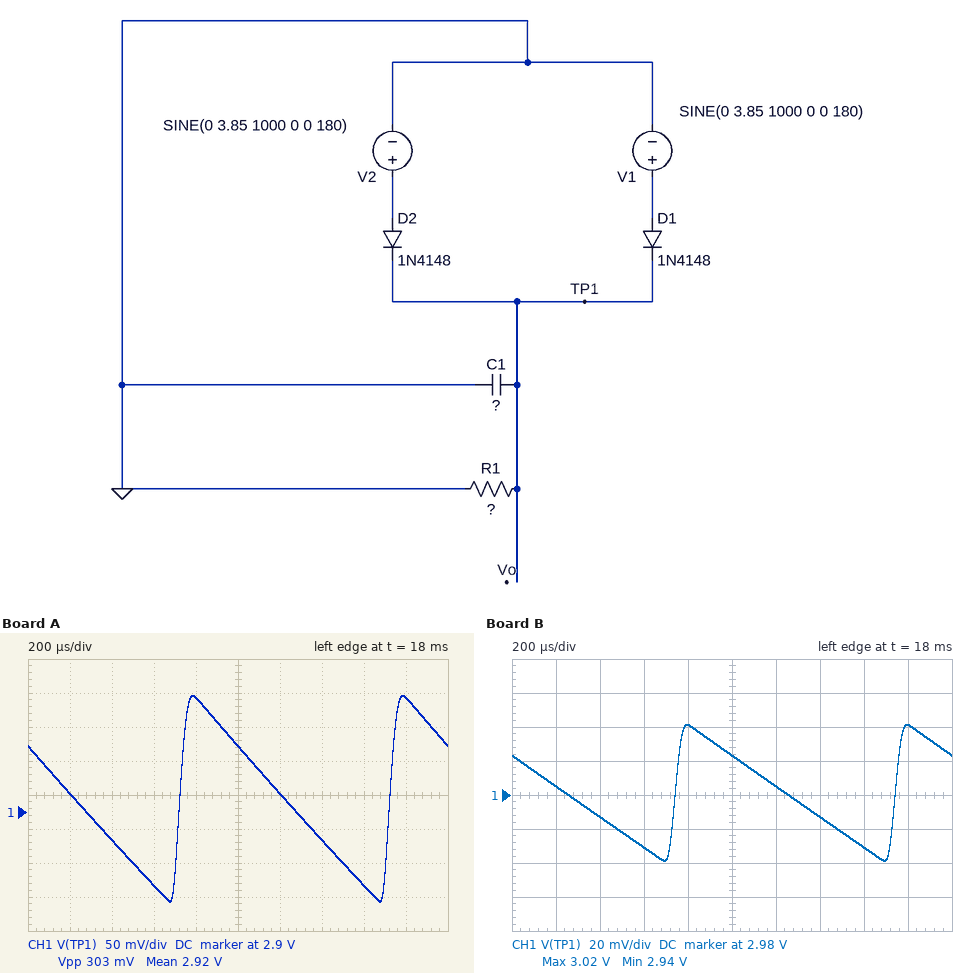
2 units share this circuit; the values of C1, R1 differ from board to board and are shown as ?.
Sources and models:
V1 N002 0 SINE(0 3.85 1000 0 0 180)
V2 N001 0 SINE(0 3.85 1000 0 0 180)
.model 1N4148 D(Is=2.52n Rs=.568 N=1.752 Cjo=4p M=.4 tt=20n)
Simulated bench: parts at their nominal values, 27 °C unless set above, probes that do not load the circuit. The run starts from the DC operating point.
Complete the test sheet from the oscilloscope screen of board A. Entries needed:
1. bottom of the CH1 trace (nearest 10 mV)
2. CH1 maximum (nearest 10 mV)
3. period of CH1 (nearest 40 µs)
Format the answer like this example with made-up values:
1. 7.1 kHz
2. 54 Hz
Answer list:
1. 2.77 V
2. 3.07 V
3. 1.00 ms
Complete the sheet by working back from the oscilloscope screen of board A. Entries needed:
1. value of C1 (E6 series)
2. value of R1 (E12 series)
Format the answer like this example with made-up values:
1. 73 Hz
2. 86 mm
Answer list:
1. 47 µF
2. 180 Ω
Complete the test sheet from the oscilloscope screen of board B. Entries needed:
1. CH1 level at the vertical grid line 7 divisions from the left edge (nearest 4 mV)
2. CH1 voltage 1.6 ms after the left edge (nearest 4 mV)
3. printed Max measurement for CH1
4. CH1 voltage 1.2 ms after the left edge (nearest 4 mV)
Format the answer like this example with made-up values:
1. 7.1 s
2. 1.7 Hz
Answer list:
1. 2.968 V
2. 2.948 V
3. 3.02 V
4. 2.984 V
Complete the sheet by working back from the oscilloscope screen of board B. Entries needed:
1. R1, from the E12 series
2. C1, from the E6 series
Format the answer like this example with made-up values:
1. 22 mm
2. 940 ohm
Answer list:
1. 220 Ω
2. 150 µF
